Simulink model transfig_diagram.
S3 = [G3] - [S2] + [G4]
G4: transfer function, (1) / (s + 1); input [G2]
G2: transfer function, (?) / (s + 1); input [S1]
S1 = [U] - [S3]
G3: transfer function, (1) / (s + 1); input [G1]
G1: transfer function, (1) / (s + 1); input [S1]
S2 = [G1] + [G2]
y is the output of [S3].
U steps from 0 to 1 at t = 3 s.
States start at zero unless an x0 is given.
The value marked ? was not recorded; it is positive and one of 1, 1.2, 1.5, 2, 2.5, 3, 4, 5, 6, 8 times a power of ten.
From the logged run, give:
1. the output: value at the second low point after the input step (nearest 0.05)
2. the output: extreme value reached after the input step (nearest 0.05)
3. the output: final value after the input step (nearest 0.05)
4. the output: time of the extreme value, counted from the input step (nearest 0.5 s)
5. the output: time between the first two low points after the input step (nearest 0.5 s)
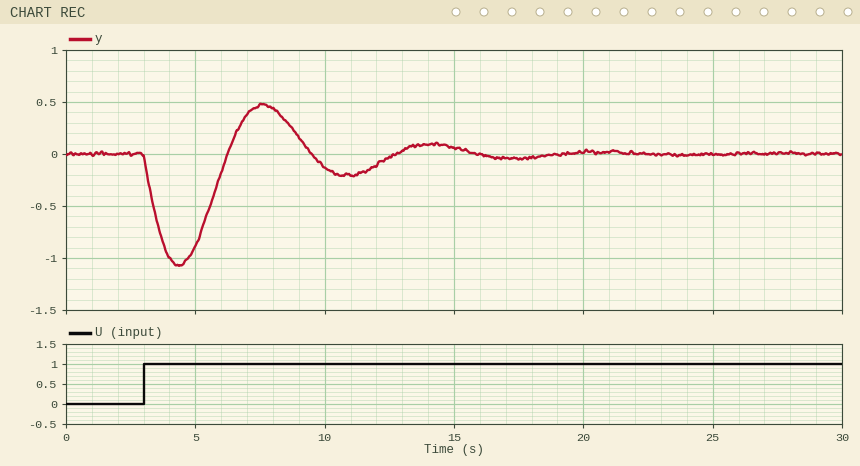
-0.20
-1.05
0.00
1.5 s
6.5 s
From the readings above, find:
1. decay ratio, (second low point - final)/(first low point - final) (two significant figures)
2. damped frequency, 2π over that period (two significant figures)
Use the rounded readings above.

0.19
0.97 rad/s
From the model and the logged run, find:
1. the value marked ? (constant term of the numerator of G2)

0.5
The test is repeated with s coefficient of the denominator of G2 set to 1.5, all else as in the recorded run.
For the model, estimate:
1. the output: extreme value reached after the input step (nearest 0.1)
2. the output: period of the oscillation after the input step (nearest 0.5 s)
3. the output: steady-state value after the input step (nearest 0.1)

-0.9
7.0 s
0.0
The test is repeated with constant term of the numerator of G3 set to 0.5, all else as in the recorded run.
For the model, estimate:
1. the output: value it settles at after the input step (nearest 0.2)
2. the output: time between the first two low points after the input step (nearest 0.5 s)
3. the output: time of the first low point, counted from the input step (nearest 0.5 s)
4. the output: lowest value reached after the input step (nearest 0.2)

-1.0
9.5 s
2.5 s
-2.0
